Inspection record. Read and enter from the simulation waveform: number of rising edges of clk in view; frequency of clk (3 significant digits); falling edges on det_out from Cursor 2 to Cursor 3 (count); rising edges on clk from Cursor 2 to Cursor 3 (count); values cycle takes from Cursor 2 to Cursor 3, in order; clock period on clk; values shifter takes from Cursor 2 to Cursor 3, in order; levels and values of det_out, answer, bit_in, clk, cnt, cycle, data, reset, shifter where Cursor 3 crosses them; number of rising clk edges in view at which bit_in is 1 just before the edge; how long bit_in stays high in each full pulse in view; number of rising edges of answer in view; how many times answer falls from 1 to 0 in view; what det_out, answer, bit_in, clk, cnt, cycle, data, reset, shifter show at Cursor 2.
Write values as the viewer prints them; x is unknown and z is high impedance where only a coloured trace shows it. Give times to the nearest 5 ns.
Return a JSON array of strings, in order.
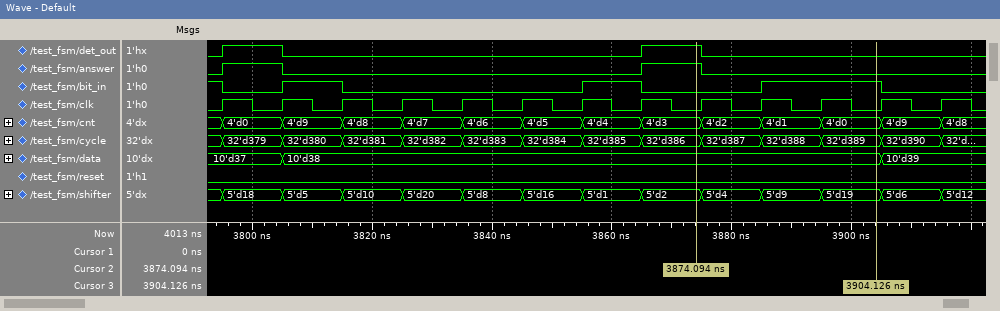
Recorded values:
["13", "100 MHz", "1", "3", "32'd386, 32'd387, 32'd388, 32'd389", "10 ns", "5'd2, 5'd4, 5'd9, 5'd19", "det_out=0, answer=0, bit_in=1, clk=0, cnt=4'd0, cycle=32'd389, data=10'd38, reset=0, shifter=5'd19", "5", "10 ns, 10 ns, 20 ns", "2", "2", "det_out=1, answer=1, bit_in=0, clk=0, cnt=4'd3, cycle=32'd386, data=10'd38, reset=0, shifter=5'd2"]
